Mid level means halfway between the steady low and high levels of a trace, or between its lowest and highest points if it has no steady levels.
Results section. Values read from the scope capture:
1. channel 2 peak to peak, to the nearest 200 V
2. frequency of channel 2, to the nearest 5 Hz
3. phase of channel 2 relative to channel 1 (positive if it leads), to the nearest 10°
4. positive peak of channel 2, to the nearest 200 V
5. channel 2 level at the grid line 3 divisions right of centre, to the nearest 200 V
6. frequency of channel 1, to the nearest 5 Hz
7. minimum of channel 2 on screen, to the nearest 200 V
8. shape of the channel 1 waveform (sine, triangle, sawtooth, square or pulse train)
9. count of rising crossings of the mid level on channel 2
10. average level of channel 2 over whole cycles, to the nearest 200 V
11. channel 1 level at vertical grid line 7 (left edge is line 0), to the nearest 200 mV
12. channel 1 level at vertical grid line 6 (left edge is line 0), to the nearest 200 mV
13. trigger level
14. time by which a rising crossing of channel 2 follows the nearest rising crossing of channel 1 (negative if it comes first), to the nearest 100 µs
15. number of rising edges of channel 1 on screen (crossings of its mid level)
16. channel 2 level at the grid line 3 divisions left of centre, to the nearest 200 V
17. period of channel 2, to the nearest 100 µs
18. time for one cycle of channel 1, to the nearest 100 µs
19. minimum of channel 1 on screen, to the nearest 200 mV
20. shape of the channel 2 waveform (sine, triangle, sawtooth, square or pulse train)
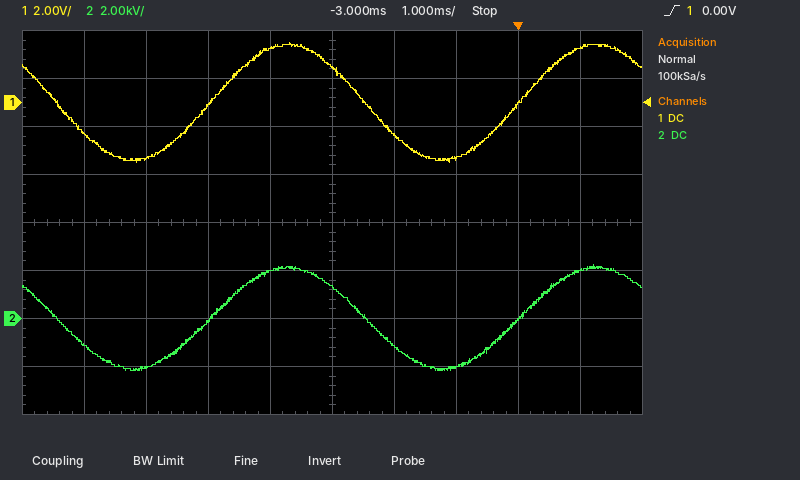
4.4 kV
200 Hz
0°
2.2 kV
0.0 kV
200 Hz
-2.2 kV
sine
2
0.0 kV
-2.4 V
-1.4 V
0.00 V
0.0 ms
2
-2.0 kV
5.0 ms
5.0 ms
-2.4 V
sine
